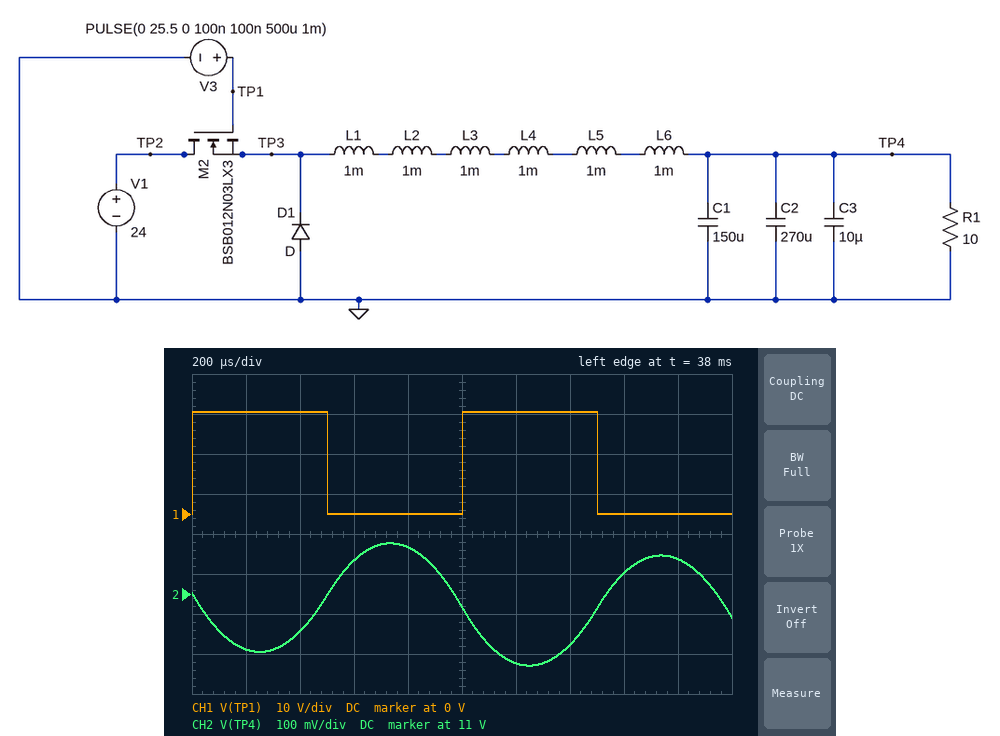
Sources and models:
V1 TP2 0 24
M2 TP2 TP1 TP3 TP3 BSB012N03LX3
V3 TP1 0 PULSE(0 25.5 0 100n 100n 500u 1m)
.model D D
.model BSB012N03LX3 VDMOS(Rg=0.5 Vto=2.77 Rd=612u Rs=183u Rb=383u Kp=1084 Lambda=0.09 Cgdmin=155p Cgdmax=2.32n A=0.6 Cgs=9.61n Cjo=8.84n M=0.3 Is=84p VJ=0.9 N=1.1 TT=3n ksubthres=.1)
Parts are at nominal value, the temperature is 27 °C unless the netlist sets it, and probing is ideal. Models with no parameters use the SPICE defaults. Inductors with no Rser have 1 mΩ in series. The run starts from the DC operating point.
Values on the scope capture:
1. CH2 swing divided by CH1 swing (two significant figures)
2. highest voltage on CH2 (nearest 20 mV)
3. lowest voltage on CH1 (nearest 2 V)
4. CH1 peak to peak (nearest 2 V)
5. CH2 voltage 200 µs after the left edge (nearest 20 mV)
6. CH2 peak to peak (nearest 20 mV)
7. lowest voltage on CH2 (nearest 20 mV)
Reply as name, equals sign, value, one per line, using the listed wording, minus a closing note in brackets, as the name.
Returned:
CH2 swing divided by CH1 swing = 0.012
highest voltage on CH2 = 11.12 V
lowest voltage on CH1 = 0 V
CH1 peak to peak = 26 V
CH2 voltage 200 µs after the left edge = 10.86 V
CH2 peak to peak = 300 mV
lowest voltage on CH2 = 10.82 V
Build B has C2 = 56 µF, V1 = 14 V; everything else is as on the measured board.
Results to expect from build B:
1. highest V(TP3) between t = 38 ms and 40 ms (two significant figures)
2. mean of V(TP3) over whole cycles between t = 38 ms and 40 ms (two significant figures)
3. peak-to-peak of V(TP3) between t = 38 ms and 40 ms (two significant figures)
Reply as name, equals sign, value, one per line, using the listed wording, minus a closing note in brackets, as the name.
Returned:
highest V(TP3) between t = 38 ms and 40 ms = 14 V
mean of V(TP3) over whole cycles between t = 38 ms and 40 ms = 6.6 V
peak-to-peak of V(TP3) between t = 38 ms and 40 ms = 15 V
